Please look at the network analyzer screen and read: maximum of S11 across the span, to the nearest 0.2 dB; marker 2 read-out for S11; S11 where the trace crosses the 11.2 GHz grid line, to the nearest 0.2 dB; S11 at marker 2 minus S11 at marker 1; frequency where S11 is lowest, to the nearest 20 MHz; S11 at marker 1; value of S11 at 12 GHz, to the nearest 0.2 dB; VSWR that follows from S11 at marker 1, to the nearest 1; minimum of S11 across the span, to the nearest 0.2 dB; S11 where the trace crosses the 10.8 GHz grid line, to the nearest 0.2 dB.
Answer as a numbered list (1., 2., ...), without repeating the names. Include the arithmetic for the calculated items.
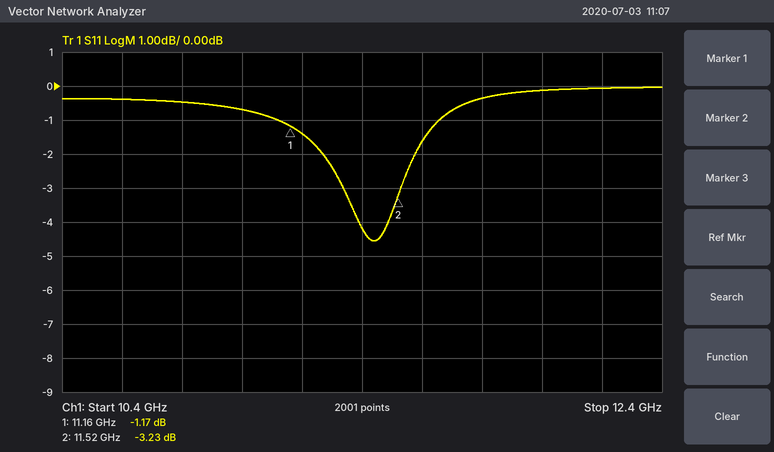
1. 0.0 dB
2. -3.23 dB
3. -1.4 dB
4. -3.23 − (-1.17) = -2.06 dB
5. 11.44 GHz
6. -1.17 dB
7. -0.2 dB
8. (1 + 0.8740)/(1 − 0.8740) ≈ 15
9. -4.6 dB
10. -0.4 dB
